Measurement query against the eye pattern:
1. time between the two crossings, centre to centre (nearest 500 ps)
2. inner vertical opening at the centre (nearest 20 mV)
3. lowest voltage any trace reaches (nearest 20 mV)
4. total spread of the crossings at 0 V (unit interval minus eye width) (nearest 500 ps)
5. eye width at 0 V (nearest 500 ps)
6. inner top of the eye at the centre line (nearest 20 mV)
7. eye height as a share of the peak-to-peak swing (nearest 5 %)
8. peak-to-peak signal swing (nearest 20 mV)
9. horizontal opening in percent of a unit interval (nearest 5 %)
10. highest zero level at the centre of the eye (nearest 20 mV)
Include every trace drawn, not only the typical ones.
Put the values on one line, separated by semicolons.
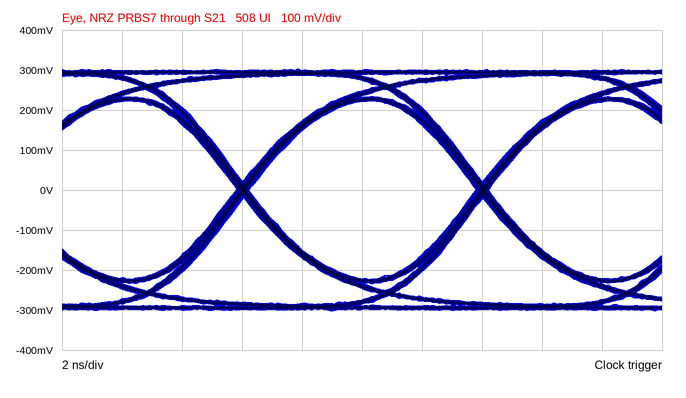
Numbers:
8.0 ns; 440 mV; -300 mV; 500 ps; 7.5 ns; 220 mV; 75 %; 600 mV; 95 %; -220 mV
